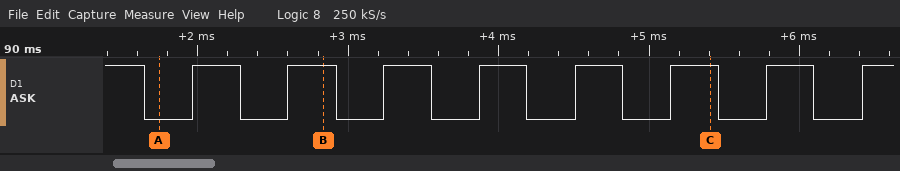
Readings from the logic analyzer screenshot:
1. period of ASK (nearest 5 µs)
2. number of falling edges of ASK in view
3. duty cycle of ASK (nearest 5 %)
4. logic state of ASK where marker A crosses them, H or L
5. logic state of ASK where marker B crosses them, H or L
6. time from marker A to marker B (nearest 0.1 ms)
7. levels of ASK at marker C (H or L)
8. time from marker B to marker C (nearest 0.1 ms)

635 µs
8
50 %
ASK=L
ASK=H
1.1 ms
ASK=H
2.6 ms
